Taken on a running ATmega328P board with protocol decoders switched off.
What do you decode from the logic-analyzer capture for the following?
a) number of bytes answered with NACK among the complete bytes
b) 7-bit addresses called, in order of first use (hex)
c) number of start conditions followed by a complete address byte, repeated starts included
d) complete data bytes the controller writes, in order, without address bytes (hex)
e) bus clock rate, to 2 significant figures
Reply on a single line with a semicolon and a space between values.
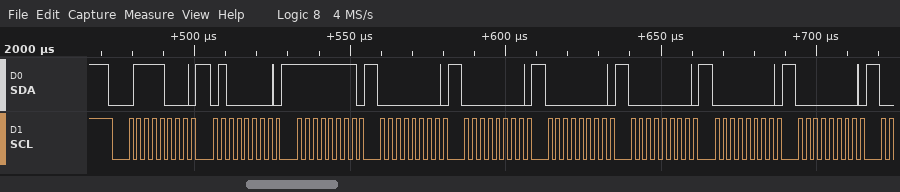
0; 0x3C; 1; 40 FF 00 00 00 00 00 00; 400 kHz
